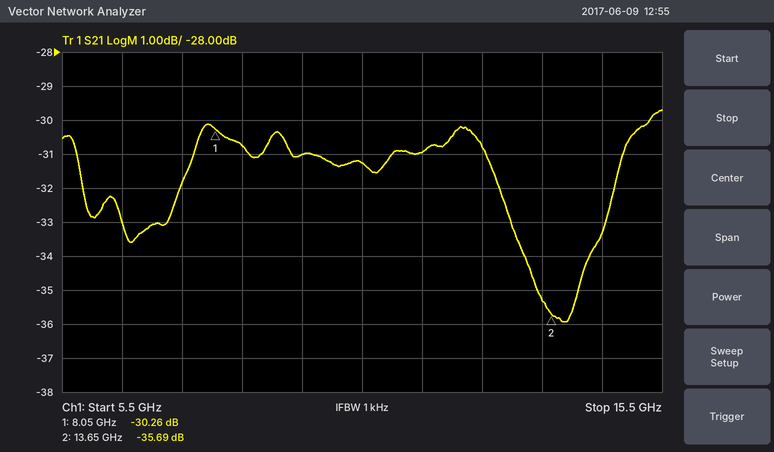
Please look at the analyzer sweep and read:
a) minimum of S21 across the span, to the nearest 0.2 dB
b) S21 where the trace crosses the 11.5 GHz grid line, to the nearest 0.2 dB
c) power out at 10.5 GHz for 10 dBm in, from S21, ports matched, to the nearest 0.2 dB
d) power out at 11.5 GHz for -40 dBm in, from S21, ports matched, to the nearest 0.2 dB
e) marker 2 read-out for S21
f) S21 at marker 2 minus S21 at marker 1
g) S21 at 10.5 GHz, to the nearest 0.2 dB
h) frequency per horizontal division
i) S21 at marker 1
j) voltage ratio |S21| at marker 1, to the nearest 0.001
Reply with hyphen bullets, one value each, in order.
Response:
- -36.0 dB
- -31.0 dB
- -21.2 dBm
- -71.0 dBm
- -35.69 dB
- -5.43 dB
- -31.2 dB
- 1 GHz
- -30.26 dB
- 0.031
